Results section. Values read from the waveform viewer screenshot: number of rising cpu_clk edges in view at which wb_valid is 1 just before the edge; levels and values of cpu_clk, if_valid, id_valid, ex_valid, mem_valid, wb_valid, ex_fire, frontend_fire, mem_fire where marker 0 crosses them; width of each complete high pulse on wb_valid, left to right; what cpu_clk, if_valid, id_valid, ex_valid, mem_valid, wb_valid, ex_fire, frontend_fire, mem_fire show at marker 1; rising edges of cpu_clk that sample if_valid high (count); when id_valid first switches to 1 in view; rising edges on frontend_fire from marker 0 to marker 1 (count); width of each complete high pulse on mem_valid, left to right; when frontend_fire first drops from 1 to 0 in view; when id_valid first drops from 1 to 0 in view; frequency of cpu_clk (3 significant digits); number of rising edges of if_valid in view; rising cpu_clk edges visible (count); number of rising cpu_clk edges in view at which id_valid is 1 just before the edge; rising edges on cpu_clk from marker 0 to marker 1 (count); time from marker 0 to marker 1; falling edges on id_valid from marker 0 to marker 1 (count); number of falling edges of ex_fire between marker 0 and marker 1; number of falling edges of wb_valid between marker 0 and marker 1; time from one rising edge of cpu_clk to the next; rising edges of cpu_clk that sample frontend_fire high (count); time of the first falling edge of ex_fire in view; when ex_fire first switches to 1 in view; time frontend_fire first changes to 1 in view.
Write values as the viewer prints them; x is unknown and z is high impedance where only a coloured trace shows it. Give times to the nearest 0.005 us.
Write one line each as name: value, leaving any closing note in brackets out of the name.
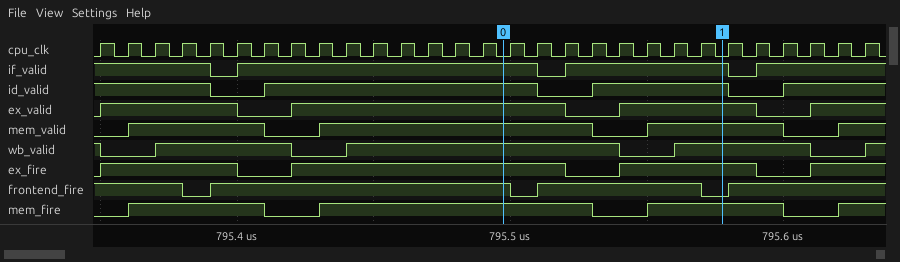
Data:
number of rising cpu_clk edges in view at which wb_valid is 1 just before the edge: 21
levels and values of cpu_clk, if_valid, id_valid, ex_valid, mem_valid, wb_valid, ex_fire, frontend_fire, mem_fire where marker 0 crosses them: cpu_clk=0, if_valid=1, id_valid=1, ex_valid=1, mem_valid=1, wb_valid=1, ex_fire=1, frontend_fire=1, mem_fire=1
width of each complete high pulse on wb_valid, left to right: 0.05 us, 0.1 us, 0.05 us
what cpu_clk, if_valid, id_valid, ex_valid, mem_valid, wb_valid, ex_fire, frontend_fire, mem_fire show at marker 1: cpu_clk=0, if_valid=1, id_valid=1, ex_valid=1, mem_valid=1, wb_valid=1, ex_fire=1, frontend_fire=0, mem_fire=1
rising edges of cpu_clk that sample if_valid high: 26
when id_valid first switches to 1 in view: 795.41 us
rising edges on frontend_fire from marker 0 to marker 1: 1
width of each complete high pulse on mem_valid, left to right: 0.05 us, 0.1 us, 0.05 us
when frontend_fire first drops from 1 to 0 in view: 795.38 us
when id_valid first drops from 1 to 0 in view: 795.39 us
frequency of cpu_clk: 100 MHz
number of rising edges of if_valid in view: 3
rising cpu_clk edges visible: 29
number of rising cpu_clk edges in view at which id_valid is 1 just before the edge: 23
rising edges on cpu_clk from marker 0 to marker 1: 8
time from marker 0 to marker 1: 0.08 us
falling edges on id_valid from marker 0 to marker 1: 1
number of falling edges of ex_fire between marker 0 and marker 1: 1
number of falling edges of wb_valid between marker 0 and marker 1: 1
time from one rising edge of cpu_clk to the next: 0.01 us
rising edges of cpu_clk that sample frontend_fire high: 26
time of the first falling edge of ex_fire in view: 795.4 us
when ex_fire first switches to 1 in view: 795.35 us
time frontend_fire first changes to 1 in view: 795.39 us
